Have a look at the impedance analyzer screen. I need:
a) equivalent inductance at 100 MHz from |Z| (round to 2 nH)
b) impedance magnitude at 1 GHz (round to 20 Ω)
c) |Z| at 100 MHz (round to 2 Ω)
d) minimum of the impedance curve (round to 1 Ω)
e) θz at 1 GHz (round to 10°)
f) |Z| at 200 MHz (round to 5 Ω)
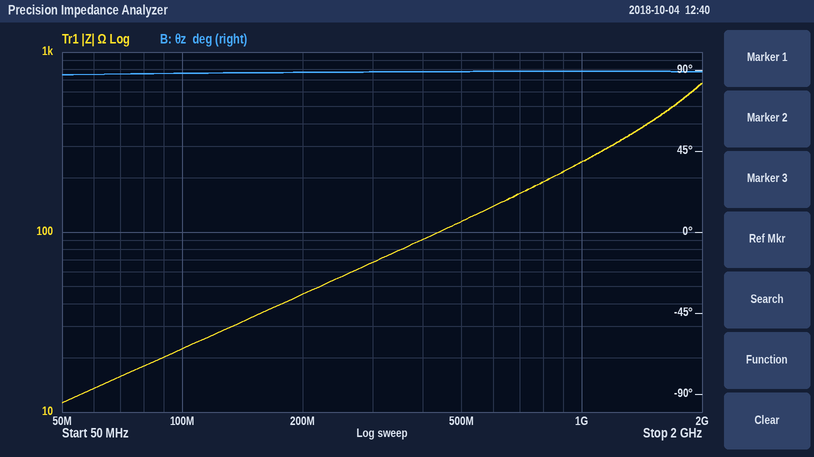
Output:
36 nH
240 Ω
22 Ω
11 Ω
90°
45 Ω
